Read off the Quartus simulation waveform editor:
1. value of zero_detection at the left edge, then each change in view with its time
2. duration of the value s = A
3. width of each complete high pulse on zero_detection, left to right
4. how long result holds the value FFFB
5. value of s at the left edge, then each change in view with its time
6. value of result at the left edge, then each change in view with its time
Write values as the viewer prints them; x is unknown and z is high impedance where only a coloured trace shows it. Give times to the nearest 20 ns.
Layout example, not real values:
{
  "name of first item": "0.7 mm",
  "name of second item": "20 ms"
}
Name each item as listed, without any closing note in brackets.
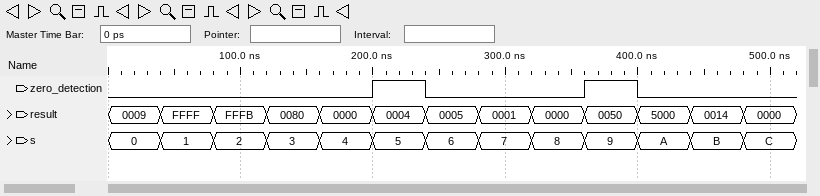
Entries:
{
  "value of zero_detection at the left edge, then each change in view with its time": "0, 1 at 200 ns, 0 at 240 ns, 1 at 360 ns, 0 at 400 ns",
  "duration of the value s = A": "40 ns",
  "width of each complete high pulse on zero_detection, left to right": "40 ns, 40 ns",
  "how long result holds the value FFFB": "40 ns",
  "value of s at the left edge, then each change in view with its time": "0, 1 at 40 ns, 2 at 80 ns, 3 at 120 ns, 4 at 160 ns, 5 at 200 ns, 6 at 240 ns, 7 at 280 ns, 8 at 320 ns, 9 at 360 ns, A at 400 ns, B at 440 ns, C at 480 ns",
  "value of result at the left edge, then each change in view with its time": "0009, FFFF at 40 ns, FFFB at 80 ns, 0080 at 120 ns, 0000 at 160 ns, 0004 at 200 ns, 0005 at 240 ns, 0001 at 280 ns, 0000 at 320 ns, 0050 at 360 ns, 5000 at 400 ns, 0014 at 440 ns, 0000 at 480 ns"
}
